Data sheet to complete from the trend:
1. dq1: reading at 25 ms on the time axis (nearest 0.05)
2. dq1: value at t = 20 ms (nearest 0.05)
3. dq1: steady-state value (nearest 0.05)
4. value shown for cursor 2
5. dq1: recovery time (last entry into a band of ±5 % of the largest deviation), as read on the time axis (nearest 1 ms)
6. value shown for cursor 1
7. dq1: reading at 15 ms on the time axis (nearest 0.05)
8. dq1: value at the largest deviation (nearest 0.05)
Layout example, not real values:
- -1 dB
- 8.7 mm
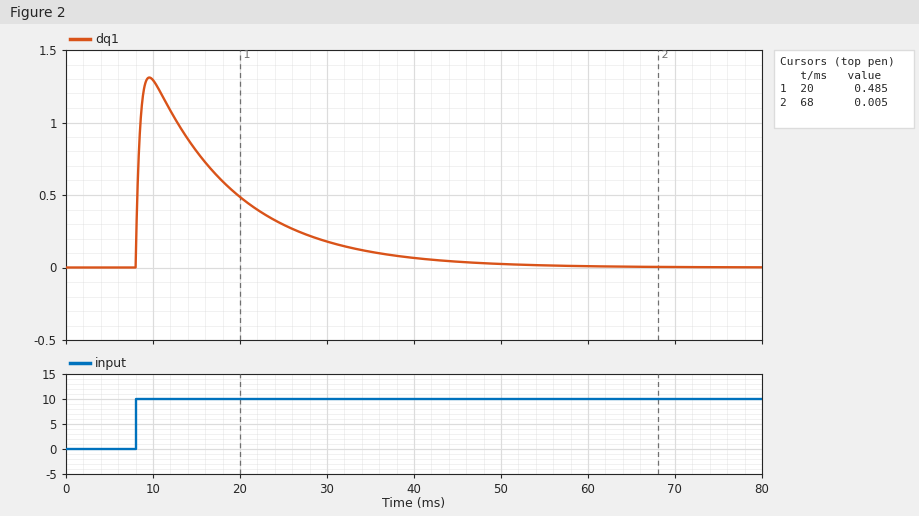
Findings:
- 0.30
- 0.50
- 0.00
- 0.005
- 40 ms
- 0.485
- 0.80
- 1.30
